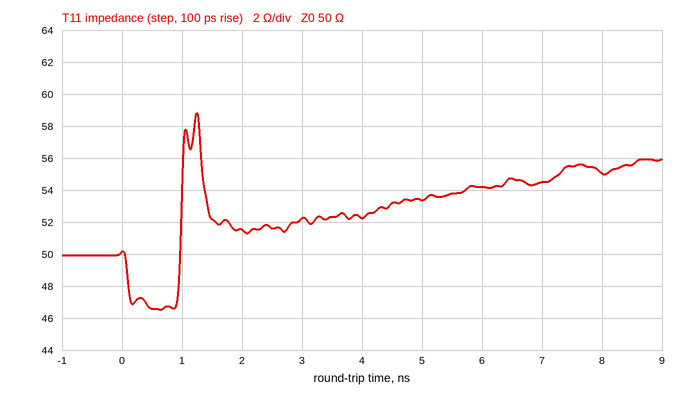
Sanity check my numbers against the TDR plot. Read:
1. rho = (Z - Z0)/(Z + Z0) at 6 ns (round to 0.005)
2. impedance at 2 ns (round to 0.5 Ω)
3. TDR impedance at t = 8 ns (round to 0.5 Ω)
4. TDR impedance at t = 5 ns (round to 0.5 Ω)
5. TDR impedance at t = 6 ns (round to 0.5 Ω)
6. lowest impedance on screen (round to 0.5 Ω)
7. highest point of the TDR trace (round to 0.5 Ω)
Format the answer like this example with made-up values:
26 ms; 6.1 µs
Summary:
+0.040; 51.5 Ω; 55.0 Ω; 53.5 Ω; 54.0 Ω; 46.5 Ω; 59.0 Ω
